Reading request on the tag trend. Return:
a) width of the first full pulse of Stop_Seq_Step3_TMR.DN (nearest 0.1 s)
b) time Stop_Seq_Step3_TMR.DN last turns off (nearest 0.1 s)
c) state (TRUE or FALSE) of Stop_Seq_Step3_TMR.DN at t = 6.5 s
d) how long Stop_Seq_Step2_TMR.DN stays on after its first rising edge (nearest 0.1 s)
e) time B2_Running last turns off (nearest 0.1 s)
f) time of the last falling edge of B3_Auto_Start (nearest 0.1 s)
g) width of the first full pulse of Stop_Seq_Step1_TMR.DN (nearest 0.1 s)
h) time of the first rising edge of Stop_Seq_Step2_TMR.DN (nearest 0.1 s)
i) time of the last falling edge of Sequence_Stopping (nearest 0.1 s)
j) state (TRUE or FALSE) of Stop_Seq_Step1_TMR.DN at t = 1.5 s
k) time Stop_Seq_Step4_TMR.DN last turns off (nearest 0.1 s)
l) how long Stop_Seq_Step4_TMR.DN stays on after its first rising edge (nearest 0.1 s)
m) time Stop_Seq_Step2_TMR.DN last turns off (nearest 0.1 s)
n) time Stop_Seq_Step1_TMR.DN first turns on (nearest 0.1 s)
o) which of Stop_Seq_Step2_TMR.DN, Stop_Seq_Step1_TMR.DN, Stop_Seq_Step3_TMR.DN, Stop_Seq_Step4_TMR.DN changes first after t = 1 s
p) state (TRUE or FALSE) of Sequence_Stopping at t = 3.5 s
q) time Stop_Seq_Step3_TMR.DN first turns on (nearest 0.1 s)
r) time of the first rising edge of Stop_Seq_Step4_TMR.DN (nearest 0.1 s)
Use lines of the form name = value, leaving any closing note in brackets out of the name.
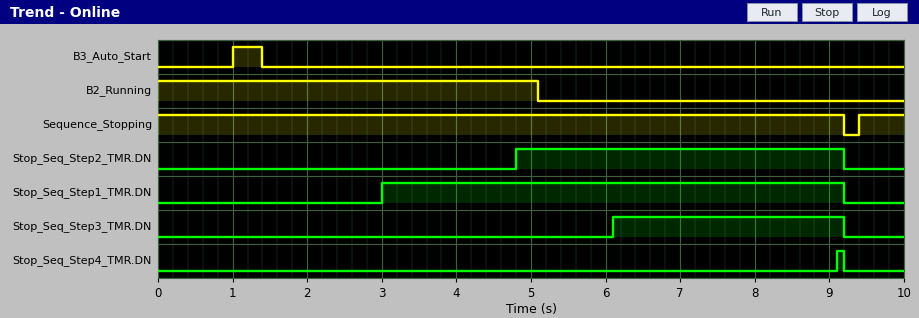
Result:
width of the first full pulse of Stop_Seq_Step3_TMR.DN = 3.1 s
time Stop_Seq_Step3_TMR.DN last turns off = 9.2 s
state (TRUE or FALSE) of Stop_Seq_Step3_TMR.DN at t = 6.5 s = TRUE
how long Stop_Seq_Step2_TMR.DN stays on after its first rising edge = 4.4 s
time B2_Running last turns off = 5.1 s
time of the last falling edge of B3_Auto_Start = 1.4 s
width of the first full pulse of Stop_Seq_Step1_TMR.DN = 6.2 s
time of the first rising edge of Stop_Seq_Step2_TMR.DN = 4.8 s
time of the last falling edge of Sequence_Stopping = 9.2 s
state (TRUE or FALSE) of Stop_Seq_Step1_TMR.DN at t = 1.5 s = FALSE
time Stop_Seq_Step4_TMR.DN last turns off = 9.2 s
how long Stop_Seq_Step4_TMR.DN stays on after its first rising edge = 0.1 s
time Stop_Seq_Step2_TMR.DN last turns off = 9.2 s
time Stop_Seq_Step1_TMR.DN first turns on = 3.0 s
which of Stop_Seq_Step2_TMR.DN, Stop_Seq_Step1_TMR.DN, Stop_Seq_Step3_TMR.DN, Stop_Seq_Step4_TMR.DN changes first after t = 1 s = Stop_Seq_Step1_TMR.DN
state (TRUE or FALSE) of Sequence_Stopping at t = 3.5 s = TRUE
time Stop_Seq_Step3_TMR.DN first turns on = 6.1 s
time of the first rising edge of Stop_Seq_Step4_TMR.DN = 9.1 s
